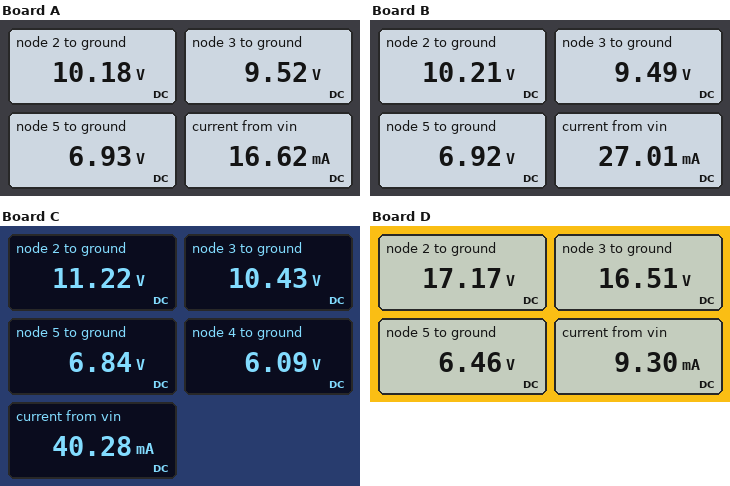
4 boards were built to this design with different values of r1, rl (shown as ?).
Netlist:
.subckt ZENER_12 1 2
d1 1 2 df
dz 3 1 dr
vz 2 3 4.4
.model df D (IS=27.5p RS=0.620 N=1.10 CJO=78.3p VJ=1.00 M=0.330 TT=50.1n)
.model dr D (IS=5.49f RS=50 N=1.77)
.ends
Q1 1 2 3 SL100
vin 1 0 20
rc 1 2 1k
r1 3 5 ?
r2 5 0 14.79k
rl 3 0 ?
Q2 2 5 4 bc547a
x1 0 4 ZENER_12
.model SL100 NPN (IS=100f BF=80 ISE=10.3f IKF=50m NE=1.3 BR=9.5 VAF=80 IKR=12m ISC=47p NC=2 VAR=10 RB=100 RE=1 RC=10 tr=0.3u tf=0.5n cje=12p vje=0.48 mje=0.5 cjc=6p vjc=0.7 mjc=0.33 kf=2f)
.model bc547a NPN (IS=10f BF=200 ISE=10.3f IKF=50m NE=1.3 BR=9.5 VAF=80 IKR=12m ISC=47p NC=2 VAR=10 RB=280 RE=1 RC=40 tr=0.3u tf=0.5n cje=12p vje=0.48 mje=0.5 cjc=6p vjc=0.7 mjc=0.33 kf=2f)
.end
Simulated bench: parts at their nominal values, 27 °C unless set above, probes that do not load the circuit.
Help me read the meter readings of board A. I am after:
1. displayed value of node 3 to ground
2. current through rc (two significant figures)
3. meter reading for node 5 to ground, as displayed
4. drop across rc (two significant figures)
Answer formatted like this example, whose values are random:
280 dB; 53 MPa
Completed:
9.52 V; 9.8 mA; 6.93 V; 9.8 V
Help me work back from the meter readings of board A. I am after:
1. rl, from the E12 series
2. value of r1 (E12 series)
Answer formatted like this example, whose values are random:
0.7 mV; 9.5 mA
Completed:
1.5 kΩ; 4.7 kΩ
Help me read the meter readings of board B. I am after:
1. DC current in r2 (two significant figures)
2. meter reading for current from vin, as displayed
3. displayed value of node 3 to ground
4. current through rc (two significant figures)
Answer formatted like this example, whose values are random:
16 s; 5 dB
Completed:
470 µA; 27.01 mA; 9.49 V; 9.8 mA
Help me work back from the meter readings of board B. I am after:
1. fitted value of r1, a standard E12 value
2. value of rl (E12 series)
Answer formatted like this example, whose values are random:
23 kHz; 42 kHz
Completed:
4.7 kΩ; 560 Ω
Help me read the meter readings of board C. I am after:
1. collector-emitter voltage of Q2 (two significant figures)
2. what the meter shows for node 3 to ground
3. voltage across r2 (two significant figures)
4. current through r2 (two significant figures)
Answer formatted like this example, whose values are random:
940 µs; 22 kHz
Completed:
5.1 V; 10.43 V; 6.8 V; 460 µA
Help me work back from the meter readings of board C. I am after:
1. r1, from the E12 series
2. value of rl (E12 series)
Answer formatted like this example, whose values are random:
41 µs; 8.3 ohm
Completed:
6.8 kΩ; 330 Ω
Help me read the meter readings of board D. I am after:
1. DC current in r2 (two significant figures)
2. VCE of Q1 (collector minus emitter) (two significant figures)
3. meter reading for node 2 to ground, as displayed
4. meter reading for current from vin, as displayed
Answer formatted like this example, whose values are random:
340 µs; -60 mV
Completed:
440 µA; 3.5 V; 17.17 V; 9.30 mA
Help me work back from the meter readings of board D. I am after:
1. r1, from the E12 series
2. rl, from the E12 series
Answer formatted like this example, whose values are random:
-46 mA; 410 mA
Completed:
22 kΩ; 2.7 kΩ
